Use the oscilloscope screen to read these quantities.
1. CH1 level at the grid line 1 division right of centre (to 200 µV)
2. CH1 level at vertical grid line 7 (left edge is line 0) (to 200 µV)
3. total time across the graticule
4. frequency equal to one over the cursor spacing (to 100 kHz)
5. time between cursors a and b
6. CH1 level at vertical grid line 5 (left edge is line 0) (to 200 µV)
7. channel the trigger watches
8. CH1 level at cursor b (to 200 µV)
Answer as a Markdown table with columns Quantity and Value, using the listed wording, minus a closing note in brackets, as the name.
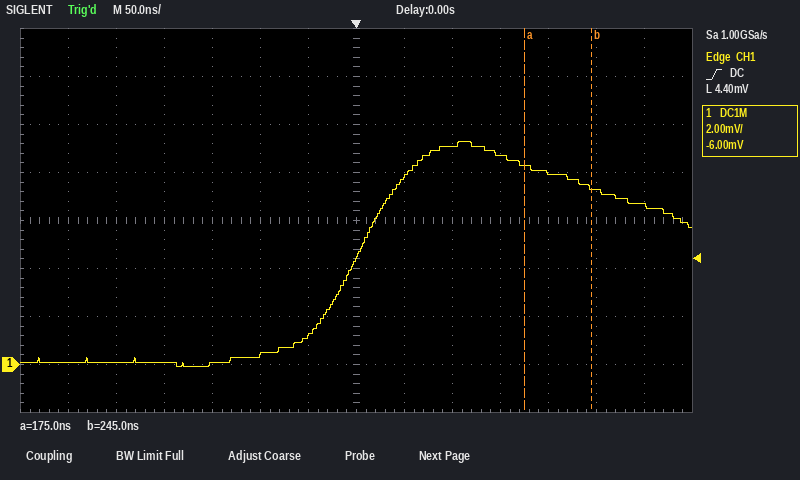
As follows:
| Quantity | Value |
|---|---|
| CH1 level at the grid line 1 division right of centre | 7.8 mV |
| CH1 level at vertical grid line 7 (left edge is line 0) | 4.4 mV |
| total time across the graticule | 700 ns |
| frequency equal to one over the cursor spacing | 14.3 MHz |
| time between cursors a and b | 70 ns |
| CH1 level at vertical grid line 5 (left edge is line 0) | 400 µV |
| channel the trigger watches | CH1 |
| CH1 level at cursor b | 7.4 mV |
